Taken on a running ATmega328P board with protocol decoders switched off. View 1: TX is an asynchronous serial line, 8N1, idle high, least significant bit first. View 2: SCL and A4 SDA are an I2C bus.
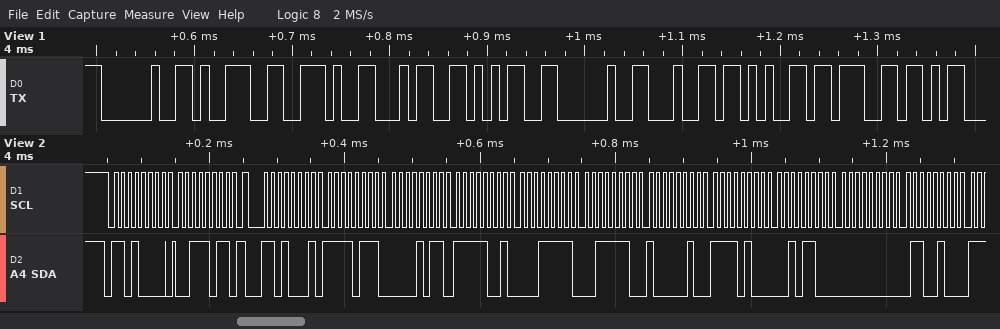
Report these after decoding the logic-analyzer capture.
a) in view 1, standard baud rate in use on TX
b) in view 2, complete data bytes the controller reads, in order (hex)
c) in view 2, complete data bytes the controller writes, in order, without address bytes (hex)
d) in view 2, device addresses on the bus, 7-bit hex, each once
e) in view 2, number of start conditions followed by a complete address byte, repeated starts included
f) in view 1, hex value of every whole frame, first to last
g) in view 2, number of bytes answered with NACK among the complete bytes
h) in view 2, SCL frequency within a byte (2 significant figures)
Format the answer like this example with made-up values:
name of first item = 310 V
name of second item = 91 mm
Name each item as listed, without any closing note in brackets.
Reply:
in view 1, standard baud rate in use on TX = 115200 baud
in view 2, complete data bytes the controller reads, in order = F7 0B F9 1F 3E 82 F4 2C 00 64
in view 2, complete data bytes the controller writes, in order, without address bytes = 3B
in view 2, device addresses on the bus, 7-bit hex, each once = 0x68
in view 2, number of start conditions followed by a complete address byte, repeated starts included = 2
in view 1, hex value of every whole frame, first to last = 20 39 2E 34 35 20 64 65 67
in view 2, number of bytes answered with NACK among the complete bytes = 0
in view 2, SCL frequency within a byte = 100 kHz
